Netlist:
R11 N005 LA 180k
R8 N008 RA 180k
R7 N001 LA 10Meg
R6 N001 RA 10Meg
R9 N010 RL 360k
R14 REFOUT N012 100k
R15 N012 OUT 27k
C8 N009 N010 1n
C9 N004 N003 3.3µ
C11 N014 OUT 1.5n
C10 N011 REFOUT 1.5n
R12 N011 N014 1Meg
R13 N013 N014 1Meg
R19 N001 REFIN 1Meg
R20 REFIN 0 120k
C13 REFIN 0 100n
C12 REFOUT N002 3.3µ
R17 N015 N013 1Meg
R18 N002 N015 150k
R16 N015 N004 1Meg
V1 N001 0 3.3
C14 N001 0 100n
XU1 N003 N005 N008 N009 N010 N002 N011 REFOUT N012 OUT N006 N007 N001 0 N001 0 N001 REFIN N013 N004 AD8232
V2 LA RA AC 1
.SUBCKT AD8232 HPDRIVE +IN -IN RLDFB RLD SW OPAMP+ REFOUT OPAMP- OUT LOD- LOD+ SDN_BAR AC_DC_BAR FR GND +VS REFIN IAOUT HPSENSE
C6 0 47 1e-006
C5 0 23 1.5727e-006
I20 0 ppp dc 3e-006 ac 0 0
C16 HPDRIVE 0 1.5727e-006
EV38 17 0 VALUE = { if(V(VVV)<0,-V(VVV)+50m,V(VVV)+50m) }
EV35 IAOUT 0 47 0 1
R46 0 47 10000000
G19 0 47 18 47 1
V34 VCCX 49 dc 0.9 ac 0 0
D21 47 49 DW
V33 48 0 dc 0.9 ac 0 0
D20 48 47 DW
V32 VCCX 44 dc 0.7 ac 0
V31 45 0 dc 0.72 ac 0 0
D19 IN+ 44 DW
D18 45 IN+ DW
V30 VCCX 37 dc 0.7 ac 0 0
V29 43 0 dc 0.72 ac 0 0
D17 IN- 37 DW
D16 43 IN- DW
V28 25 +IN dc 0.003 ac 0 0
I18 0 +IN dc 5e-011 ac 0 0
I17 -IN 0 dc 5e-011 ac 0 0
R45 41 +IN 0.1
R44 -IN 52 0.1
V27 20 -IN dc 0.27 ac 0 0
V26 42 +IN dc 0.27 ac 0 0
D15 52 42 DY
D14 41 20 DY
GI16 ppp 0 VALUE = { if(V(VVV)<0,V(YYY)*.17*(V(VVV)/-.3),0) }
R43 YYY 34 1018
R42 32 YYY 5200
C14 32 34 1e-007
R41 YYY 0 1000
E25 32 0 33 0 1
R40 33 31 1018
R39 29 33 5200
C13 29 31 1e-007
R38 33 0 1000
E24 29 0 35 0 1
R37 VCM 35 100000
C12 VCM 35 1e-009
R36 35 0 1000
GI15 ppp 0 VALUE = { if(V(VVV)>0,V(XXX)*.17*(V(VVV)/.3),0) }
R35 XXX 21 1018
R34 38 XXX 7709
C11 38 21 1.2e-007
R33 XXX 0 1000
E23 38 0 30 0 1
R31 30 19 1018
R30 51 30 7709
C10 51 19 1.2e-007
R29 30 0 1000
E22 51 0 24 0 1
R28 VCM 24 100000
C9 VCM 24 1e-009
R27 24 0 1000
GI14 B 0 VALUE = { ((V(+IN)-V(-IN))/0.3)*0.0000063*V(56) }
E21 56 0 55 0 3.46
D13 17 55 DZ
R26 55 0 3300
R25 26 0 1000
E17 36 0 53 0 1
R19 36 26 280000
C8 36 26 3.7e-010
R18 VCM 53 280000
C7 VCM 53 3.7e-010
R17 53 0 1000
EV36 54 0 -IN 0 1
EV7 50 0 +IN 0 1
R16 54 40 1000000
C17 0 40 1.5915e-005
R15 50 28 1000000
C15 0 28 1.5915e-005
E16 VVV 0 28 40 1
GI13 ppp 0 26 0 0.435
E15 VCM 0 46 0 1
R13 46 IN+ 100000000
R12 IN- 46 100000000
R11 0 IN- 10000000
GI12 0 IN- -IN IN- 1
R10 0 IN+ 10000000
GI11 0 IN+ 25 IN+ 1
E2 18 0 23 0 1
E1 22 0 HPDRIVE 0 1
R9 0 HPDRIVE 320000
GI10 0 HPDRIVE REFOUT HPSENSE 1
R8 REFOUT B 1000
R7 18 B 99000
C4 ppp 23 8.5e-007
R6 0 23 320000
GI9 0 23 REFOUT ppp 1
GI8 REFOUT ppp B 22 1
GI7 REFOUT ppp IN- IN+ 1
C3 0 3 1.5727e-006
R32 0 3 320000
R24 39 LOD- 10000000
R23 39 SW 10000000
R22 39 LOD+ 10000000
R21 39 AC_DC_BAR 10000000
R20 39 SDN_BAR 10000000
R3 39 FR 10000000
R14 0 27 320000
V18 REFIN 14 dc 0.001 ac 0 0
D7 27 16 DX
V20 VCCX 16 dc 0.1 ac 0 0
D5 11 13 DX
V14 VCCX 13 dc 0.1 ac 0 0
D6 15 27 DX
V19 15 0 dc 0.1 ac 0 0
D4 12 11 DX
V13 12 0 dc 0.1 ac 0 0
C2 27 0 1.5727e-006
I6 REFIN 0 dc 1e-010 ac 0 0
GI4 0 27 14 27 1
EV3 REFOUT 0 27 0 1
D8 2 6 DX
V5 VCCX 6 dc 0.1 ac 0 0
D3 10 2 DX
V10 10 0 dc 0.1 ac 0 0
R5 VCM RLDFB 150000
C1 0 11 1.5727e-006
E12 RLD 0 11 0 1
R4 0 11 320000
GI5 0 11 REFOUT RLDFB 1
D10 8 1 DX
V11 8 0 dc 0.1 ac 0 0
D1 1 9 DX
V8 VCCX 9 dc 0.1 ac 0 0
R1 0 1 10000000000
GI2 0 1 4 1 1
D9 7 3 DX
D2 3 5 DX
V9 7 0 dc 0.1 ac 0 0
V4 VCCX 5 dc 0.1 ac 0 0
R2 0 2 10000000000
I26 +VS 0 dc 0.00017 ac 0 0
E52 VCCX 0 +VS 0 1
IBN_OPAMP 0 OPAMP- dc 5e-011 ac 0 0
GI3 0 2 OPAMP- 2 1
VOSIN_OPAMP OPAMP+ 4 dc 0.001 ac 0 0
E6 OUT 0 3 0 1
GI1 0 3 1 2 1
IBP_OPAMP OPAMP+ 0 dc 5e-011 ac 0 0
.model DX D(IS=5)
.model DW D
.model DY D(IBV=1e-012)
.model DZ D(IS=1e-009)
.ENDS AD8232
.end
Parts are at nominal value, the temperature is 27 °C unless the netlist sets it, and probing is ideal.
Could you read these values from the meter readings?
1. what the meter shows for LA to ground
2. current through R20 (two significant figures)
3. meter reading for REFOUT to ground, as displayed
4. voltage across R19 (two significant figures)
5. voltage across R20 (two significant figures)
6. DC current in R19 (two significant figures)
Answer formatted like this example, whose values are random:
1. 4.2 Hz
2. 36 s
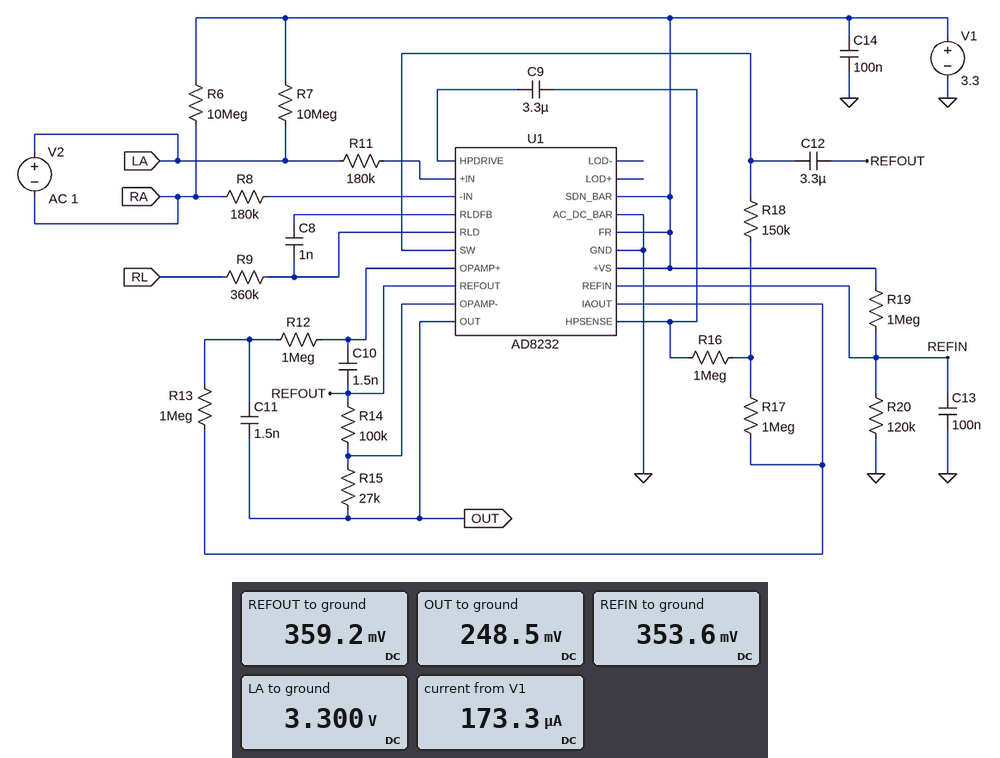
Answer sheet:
1. 3.300 V
2. 2.9 µA
3. 359.2 mV
4. 2.9 V
5. 350 mV
6. 2.9 µA
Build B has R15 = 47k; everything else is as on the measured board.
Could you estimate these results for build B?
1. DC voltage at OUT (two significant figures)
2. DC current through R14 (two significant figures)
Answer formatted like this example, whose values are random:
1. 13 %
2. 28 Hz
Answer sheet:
1. 240 mV
2. 800 nA
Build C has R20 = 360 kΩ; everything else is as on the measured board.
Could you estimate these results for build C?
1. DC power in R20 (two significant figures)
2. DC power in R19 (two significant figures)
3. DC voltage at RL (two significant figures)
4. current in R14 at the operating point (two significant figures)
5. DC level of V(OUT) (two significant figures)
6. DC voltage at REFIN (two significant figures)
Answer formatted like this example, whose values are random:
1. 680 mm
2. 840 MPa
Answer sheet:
1. 2.1 µW
2. 5.9 µW
3. 120 mV
4. 990 nA
5. 750 mV
6. 870 mV
